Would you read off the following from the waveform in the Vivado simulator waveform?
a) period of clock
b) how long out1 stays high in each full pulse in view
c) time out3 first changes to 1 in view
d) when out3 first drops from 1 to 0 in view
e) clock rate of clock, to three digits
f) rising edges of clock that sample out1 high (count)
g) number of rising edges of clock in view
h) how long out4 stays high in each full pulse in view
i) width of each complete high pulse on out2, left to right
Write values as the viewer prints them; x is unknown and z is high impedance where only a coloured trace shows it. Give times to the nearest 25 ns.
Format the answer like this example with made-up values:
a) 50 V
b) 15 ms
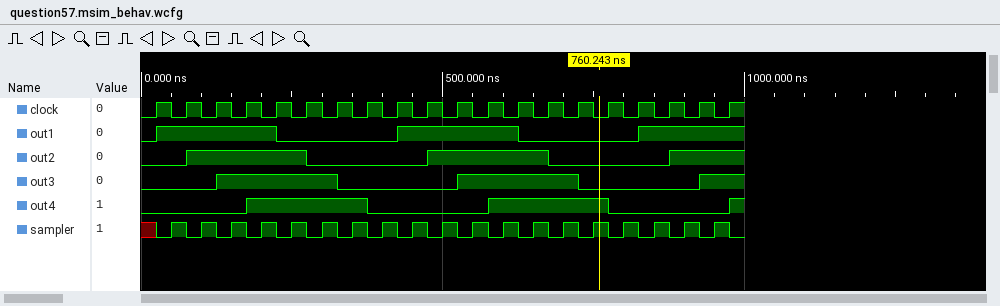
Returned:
a) 50 ns
b) 200 ns, 200 ns
c) 125 ns
d) 325 ns
e) 20.0 MHz
f) 11
g) 20
h) 200 ns, 200 ns
i) 200 ns, 200 ns
